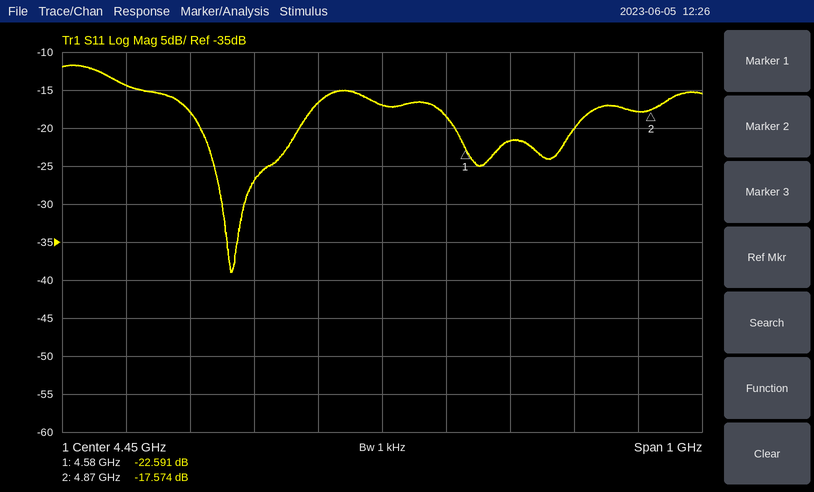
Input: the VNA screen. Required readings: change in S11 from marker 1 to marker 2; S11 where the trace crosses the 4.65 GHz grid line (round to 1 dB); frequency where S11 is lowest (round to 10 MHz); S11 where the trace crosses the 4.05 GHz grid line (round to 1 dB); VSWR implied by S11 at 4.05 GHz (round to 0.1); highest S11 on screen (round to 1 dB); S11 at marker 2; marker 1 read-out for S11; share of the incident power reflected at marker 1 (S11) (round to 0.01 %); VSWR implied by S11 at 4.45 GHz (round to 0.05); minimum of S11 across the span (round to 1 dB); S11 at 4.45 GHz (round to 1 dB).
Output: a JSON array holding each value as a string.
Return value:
["5.017 dB", "-22 dB", "4.21 GHz", "-14 dB", "1.5", "-12 dB", "-17.574 dB", "-22.591 dB", "0.55 %", "1.35", "-39 dB", "-17 dB"]
